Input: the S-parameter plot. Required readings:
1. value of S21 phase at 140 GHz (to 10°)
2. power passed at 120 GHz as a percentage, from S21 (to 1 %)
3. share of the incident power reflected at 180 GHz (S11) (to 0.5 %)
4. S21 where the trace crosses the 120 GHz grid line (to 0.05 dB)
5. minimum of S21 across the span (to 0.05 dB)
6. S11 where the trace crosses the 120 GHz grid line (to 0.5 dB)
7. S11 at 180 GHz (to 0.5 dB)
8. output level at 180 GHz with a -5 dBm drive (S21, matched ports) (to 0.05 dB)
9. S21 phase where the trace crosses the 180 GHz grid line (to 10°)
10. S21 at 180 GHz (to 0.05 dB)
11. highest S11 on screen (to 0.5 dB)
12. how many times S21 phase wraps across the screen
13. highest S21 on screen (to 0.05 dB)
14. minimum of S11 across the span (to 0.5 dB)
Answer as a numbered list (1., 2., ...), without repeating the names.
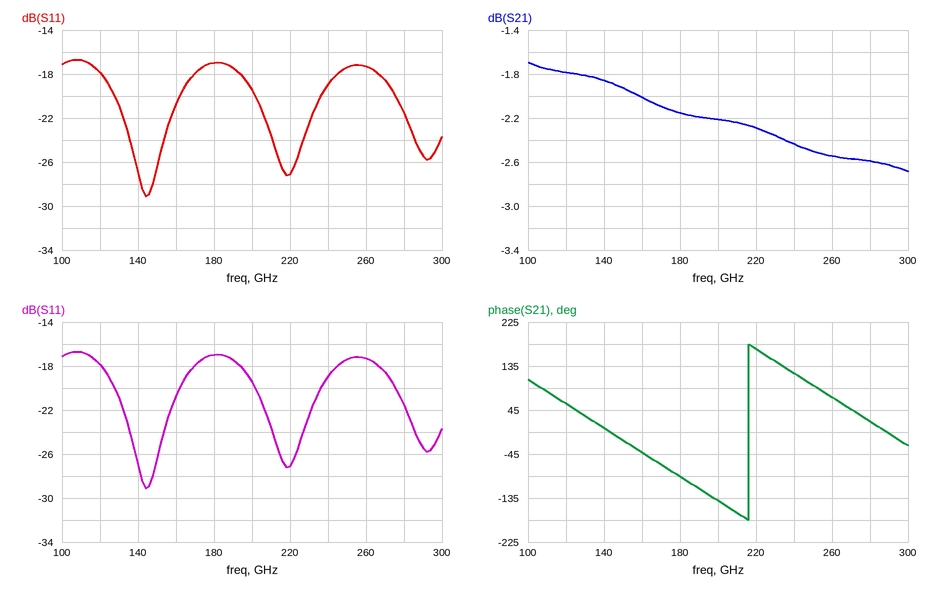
1. 10°
2. 66 %
3. 2.0 %
4. -1.80 dB
5. -2.70 dB
6. -18.0 dB
7. -17.0 dB
8. -7.15 dBm
9. -90°
10. -2.15 dB
11. -16.5 dB
12. 1
13. -1.70 dB
14. -29.0 dB
